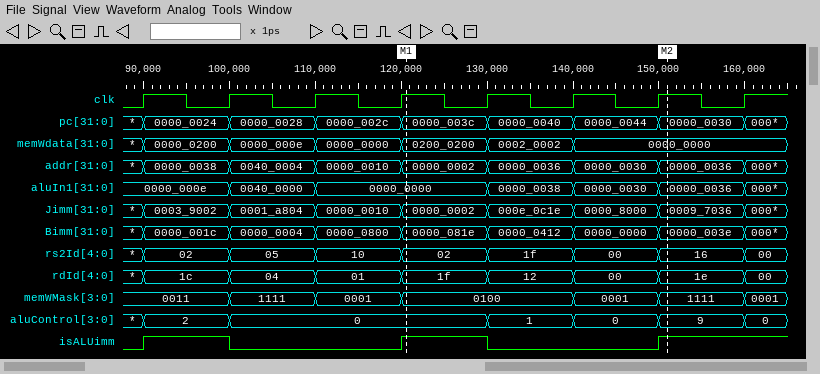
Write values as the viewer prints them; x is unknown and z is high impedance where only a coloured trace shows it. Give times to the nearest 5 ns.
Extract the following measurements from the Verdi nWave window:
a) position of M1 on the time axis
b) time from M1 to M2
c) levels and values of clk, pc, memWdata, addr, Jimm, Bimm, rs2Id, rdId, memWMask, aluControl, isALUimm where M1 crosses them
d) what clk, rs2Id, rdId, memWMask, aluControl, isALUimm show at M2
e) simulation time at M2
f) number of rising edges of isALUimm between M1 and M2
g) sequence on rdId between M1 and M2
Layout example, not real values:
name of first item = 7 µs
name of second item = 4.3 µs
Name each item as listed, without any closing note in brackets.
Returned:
position of M1 on the time axis = 120 ns
time from M1 to M2 = 30 ns
levels and values of clk, pc, memWdata, addr, Jimm, Bimm, rs2Id, rdId, memWMask, aluControl, isALUimm where M1 crosses them = clk=1, pc=0000_003c, memWdata=0200_0200, addr=0000_0002, Jimm=0000_0002, Bimm=0000_081e, rs2Id=02, rdId=1f, memWMask=0100, aluControl=0, isALUimm=1
what clk, rs2Id, rdId, memWMask, aluControl, isALUimm show at M2 = clk=1, rs2Id=16, rdId=1e, memWMask=1111, aluControl=9, isALUimm=1
simulation time at M2 = 150 ns
number of rising edges of isALUimm between M1 and M2 = 1
sequence on rdId between M1 and M2 = 1f, 12, 00, 1e
